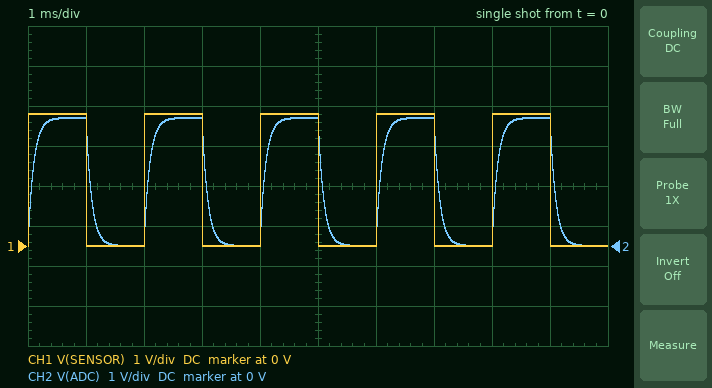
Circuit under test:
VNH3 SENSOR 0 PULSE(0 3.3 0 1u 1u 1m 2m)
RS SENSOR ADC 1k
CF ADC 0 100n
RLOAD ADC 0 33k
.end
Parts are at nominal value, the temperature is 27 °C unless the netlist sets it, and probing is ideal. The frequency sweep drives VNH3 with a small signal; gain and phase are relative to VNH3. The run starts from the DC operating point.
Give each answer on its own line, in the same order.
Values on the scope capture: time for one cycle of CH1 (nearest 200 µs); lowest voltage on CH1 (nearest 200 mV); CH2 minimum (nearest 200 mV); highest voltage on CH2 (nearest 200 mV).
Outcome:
2.0 ms
0 V
0 V
3.2 V
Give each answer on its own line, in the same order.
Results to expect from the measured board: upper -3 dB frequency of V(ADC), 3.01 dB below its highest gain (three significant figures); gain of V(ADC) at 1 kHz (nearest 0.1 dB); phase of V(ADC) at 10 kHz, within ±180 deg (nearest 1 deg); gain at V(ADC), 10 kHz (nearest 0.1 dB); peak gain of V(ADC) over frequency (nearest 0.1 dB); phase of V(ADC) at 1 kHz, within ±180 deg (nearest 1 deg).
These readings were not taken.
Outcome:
1.64 kHz
-1.6 dB
-81 deg
-16.1 dB
-0.3 dB
-31 deg
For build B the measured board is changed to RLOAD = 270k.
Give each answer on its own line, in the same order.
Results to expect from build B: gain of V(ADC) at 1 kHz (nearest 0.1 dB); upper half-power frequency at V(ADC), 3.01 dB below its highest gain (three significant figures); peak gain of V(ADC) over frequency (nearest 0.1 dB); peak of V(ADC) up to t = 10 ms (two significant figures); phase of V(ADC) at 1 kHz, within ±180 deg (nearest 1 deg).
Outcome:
-1.5 dB
1.60 kHz
0 dB
3.3 V
-32 deg
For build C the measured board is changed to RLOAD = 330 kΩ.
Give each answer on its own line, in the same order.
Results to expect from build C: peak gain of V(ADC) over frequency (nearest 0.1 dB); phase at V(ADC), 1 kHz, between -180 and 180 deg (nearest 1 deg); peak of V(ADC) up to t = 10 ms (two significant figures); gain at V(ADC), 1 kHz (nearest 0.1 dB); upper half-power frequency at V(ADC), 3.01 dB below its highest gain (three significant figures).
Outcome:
0 dB
-32 deg
3.3 V
-1.5 dB
1.60 kHz
